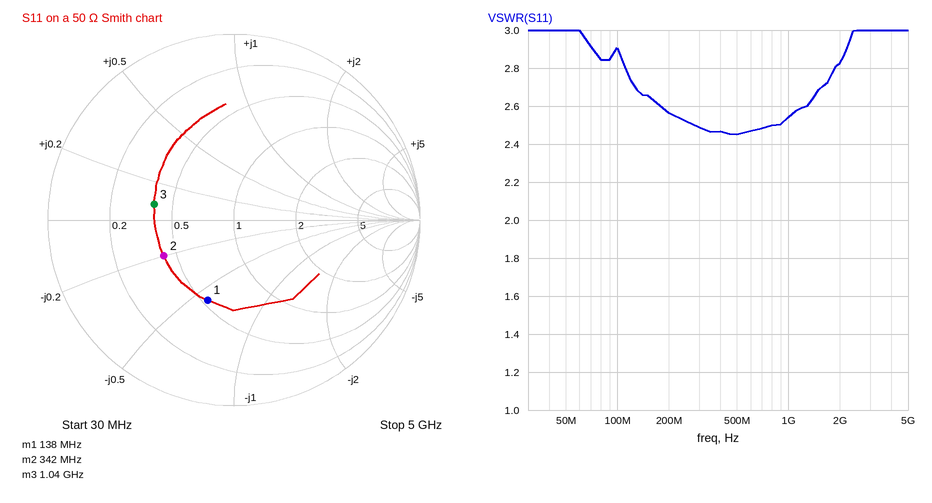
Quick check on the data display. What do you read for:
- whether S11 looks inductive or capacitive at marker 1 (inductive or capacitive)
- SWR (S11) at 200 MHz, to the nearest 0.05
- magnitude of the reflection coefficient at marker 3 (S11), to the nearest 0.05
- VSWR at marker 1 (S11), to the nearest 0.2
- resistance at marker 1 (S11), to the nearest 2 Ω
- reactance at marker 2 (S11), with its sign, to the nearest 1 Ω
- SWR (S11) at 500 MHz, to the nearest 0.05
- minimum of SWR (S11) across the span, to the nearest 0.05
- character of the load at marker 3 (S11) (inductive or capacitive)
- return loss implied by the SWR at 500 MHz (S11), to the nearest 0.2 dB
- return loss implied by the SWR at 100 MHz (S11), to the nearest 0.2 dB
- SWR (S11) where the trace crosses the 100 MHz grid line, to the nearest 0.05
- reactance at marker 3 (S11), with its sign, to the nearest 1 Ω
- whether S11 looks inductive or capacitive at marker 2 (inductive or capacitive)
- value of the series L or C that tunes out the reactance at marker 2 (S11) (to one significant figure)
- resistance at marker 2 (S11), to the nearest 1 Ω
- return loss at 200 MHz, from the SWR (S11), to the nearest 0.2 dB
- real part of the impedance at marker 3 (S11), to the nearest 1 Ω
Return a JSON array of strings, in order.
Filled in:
["capacitive", "2.55", "0.45", "2.6", "26 Ω", "-10 Ω", "2.45", "2.45", "inductive", "7.6 dB", "6.2 dB", "2.90", "+4 Ω", "capacitive", "5 nH", "21 Ω", "7.2 dB", "20 Ω"]
